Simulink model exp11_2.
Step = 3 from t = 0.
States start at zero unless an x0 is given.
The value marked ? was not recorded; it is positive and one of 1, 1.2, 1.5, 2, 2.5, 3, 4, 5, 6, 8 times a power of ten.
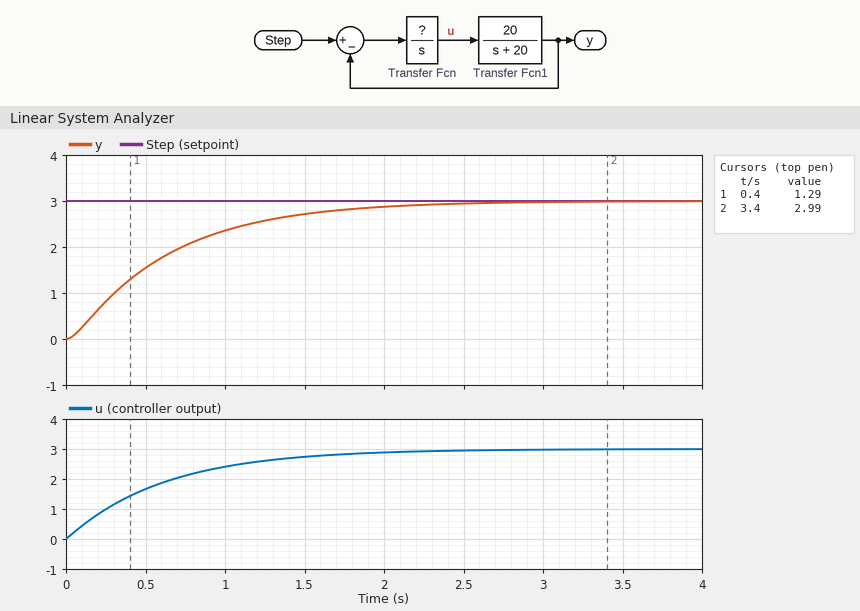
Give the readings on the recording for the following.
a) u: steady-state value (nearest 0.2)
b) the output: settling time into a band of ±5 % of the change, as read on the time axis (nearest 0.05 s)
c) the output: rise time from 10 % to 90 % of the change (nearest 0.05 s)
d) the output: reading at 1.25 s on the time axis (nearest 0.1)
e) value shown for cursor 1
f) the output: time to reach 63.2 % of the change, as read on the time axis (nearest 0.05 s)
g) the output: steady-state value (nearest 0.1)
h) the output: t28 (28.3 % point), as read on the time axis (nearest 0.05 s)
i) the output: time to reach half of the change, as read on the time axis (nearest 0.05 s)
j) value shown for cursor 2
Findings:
3.0
1.90 s
1.35 s
2.6
1.29
0.65 s
3.0
0.25 s
0.50 s
2.99
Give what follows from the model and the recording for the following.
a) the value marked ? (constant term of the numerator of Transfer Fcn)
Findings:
1.5
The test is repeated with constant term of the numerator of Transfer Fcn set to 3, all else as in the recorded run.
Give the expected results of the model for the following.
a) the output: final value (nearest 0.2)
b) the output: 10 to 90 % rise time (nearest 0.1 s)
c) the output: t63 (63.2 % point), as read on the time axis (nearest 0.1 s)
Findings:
3.0
0.6 s
0.3 s
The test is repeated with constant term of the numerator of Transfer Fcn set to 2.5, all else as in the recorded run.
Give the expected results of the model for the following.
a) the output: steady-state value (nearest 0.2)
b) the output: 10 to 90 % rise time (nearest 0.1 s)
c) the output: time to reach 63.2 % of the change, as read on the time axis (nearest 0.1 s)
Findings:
3.0
0.8 s
0.4 s
